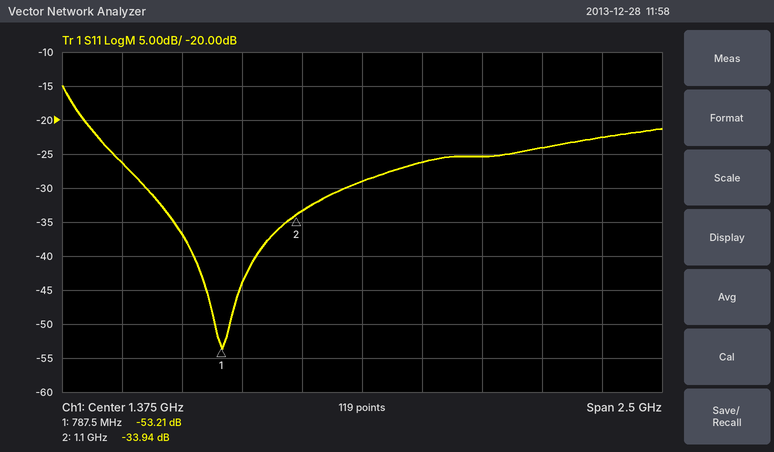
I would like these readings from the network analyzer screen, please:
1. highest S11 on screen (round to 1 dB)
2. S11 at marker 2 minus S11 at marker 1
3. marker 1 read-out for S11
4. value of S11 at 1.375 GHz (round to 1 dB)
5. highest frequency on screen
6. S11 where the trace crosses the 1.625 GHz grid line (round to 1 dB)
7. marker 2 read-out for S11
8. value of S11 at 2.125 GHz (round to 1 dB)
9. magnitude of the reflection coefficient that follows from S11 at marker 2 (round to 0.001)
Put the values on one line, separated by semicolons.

-15 dB; 19.27 dB; -53.21 dB; -29 dB; 2.625 GHz; -26 dB; -33.94 dB; -24 dB; 0.020
